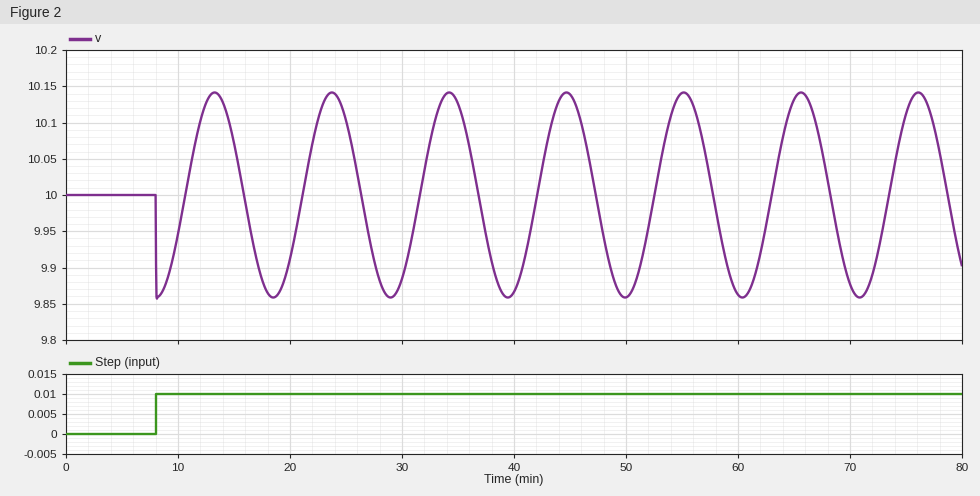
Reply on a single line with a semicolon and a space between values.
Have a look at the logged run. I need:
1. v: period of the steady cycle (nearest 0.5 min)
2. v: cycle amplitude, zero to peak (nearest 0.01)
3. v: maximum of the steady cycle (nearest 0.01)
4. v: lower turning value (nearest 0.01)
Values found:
10.5 min; 0.14; 10.14; 9.86
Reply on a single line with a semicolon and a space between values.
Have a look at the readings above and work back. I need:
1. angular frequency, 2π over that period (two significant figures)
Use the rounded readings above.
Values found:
0.60 rad/min
